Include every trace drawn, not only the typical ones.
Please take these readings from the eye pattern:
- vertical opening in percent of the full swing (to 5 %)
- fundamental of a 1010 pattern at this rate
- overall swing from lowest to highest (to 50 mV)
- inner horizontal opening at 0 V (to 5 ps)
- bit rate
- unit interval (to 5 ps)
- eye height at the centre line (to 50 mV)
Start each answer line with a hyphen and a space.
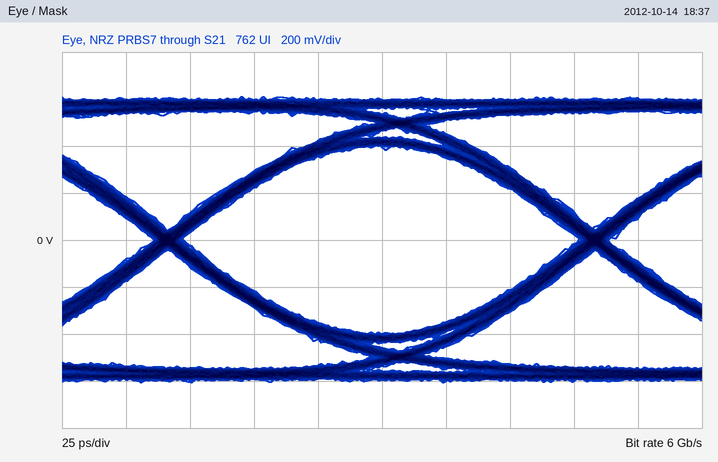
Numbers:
- 65 %
- 3 GHz
- 1.20 V
- 155 ps
- 6 Gb/s
- 165 ps
- 800 mV
